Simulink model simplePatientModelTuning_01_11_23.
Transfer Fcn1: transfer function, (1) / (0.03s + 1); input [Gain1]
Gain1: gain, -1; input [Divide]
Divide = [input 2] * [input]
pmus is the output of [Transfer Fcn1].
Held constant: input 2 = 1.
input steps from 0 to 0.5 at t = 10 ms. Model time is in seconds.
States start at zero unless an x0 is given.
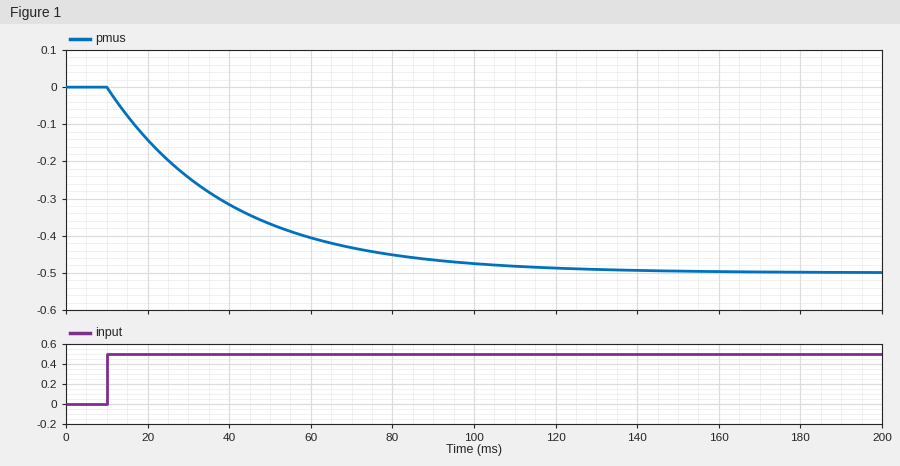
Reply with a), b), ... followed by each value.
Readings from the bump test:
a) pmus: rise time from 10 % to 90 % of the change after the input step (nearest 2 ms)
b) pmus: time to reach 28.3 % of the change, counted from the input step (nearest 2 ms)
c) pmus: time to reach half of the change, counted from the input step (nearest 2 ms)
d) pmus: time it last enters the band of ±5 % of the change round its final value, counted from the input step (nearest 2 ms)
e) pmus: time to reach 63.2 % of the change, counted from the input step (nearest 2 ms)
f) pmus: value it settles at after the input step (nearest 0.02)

a) 66 ms
b) 10 ms
c) 20 ms
d) 90 ms
e) 30 ms
f) -0.50
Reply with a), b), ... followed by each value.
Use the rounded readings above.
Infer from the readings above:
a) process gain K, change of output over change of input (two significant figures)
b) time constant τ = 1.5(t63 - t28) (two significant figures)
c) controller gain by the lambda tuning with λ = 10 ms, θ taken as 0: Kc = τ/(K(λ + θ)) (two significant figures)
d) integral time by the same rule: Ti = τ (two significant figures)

a) -1.0
b) 30 ms
c) -3.0
d) 30 ms
